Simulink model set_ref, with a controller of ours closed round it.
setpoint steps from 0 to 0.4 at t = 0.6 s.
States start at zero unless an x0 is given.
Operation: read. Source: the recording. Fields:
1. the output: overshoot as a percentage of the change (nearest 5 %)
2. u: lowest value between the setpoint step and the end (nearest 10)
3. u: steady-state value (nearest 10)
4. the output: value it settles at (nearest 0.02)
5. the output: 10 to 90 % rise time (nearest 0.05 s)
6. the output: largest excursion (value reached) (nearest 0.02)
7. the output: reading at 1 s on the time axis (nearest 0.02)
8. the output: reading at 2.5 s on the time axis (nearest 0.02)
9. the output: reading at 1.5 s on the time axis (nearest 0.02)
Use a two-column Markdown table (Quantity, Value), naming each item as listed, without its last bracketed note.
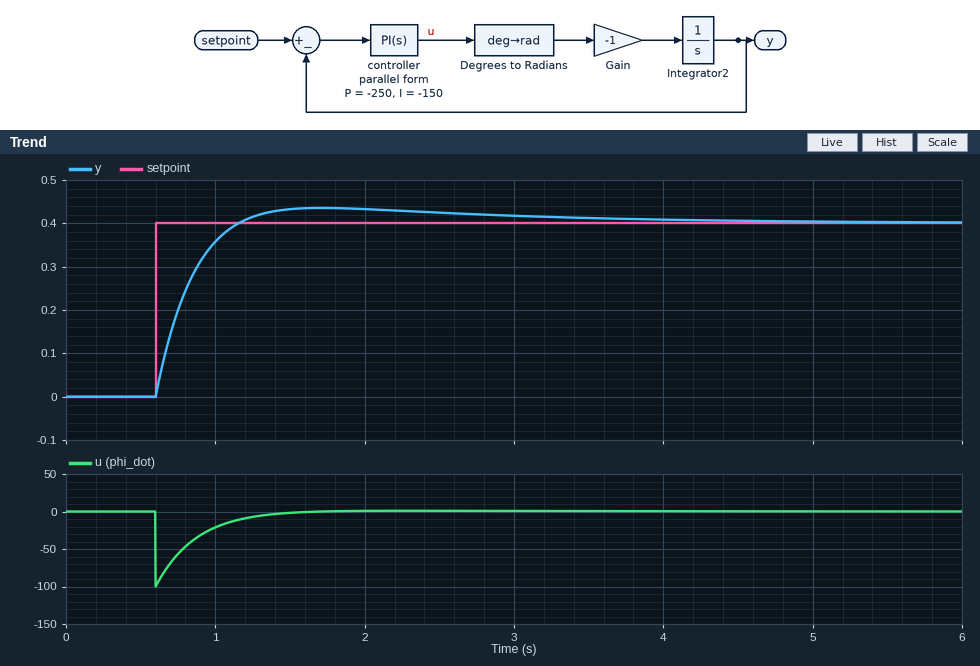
| Quantity | Value |
|---|---|
| the output: overshoot as a percentage of the change | 10 % |
| u: lowest value between the setpoint step and the end | -100 |
| u: steady-state value | 0 |
| the output: value it settles at | 0.40 |
| the output: 10 to 90 % rise time | 0.40 s |
| the output: largest excursion (value reached) | 0.44 |
| the output: reading at 1 s on the time axis | 0.36 |
| the output: reading at 2.5 s on the time axis | 0.42 |
| the output: reading at 1.5 s on the time axis | 0.44 |
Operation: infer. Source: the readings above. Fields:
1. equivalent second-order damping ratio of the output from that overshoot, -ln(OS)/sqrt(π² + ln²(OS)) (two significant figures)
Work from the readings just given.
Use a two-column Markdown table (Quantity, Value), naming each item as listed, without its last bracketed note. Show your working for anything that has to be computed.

| Quantity | Value |
|---|---|
| equivalent second-order damping ratio of the output from that overshoot, -ln(OS)/sqrt(π² + ln²(OS)) | ln(0.1) = -2.303; 2.303 / sqrt(9.870 + 5.302) = 0.59 |
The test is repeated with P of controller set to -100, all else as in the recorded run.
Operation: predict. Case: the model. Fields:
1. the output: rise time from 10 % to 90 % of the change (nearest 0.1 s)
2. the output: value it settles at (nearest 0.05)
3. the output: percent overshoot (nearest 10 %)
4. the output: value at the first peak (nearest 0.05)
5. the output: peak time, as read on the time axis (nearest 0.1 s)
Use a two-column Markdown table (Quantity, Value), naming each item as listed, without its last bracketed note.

| Quantity | Value |
|---|---|
| the output: rise time from 10 % to 90 % of the change | 0.6 s |
| the output: value it settles at | 0.40 |
| the output: percent overshoot | 30 % |
| the output: value at the first peak | 0.50 |
| the output: peak time, as read on the time axis | 2.1 s |
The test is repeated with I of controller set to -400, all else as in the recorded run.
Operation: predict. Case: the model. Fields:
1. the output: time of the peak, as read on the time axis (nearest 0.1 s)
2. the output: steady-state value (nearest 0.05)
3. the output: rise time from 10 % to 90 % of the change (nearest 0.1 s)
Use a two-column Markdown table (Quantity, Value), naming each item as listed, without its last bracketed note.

| Quantity | Value |
|---|---|
| the output: time of the peak, as read on the time axis | 1.4 s |
| the output: steady-state value | 0.40 |
| the output: rise time from 10 % to 90 % of the change | 0.3 s |
